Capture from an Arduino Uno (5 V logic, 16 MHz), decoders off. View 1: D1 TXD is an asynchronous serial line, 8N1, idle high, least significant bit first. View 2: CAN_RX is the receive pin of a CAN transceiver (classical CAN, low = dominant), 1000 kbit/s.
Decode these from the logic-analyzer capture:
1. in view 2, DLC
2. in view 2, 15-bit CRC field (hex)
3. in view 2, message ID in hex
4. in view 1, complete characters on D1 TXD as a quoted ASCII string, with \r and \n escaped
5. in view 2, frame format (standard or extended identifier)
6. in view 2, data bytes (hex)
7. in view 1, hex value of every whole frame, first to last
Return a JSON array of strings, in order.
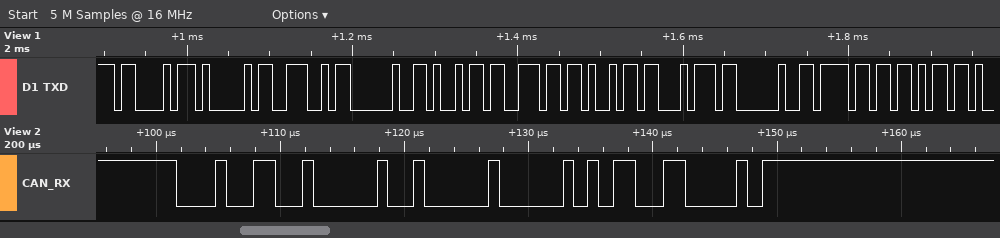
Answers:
["1", "0x0B30", "0x132", "\"CAN init ok\"", "standard", "00", "43 41 4E 20 69 6E 69 74 20 6F 6B"]
